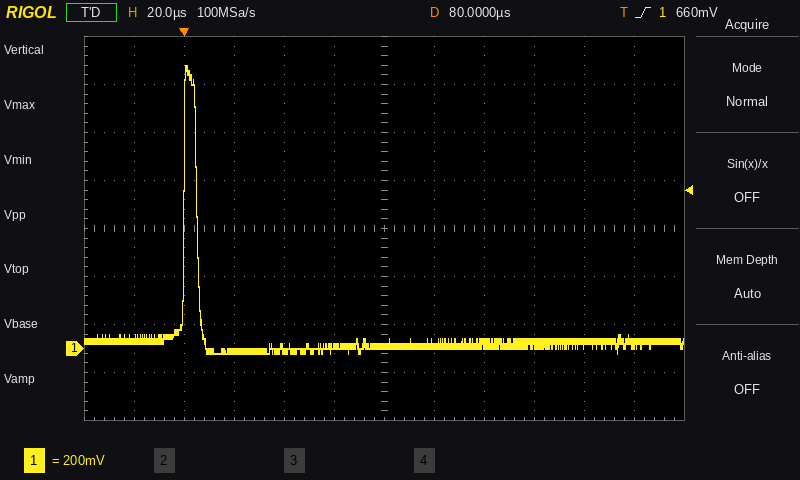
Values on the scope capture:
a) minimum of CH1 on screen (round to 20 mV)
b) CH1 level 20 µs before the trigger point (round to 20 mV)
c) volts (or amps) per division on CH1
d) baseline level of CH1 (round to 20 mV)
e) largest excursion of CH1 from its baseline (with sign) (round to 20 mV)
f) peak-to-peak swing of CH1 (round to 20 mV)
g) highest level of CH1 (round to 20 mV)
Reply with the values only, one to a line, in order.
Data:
-20 mV
40 mV
200 mV
20 mV
+1.16 V
1.20 V
1.18 V
